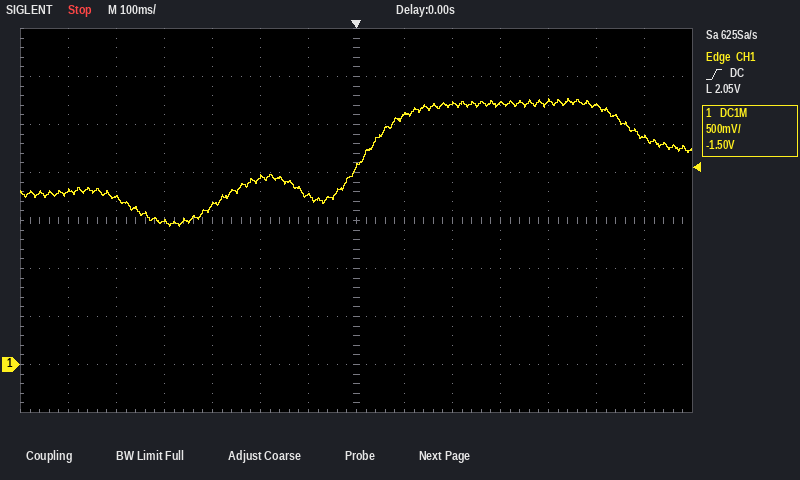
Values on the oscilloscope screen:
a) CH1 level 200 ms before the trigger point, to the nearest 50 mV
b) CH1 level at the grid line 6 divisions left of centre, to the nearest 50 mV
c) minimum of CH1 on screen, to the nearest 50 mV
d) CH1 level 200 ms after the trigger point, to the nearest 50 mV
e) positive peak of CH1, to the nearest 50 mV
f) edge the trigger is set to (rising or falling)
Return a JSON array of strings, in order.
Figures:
["1.95 V", "1.80 V", "1.45 V", "2.70 V", "2.75 V", "rising"]
